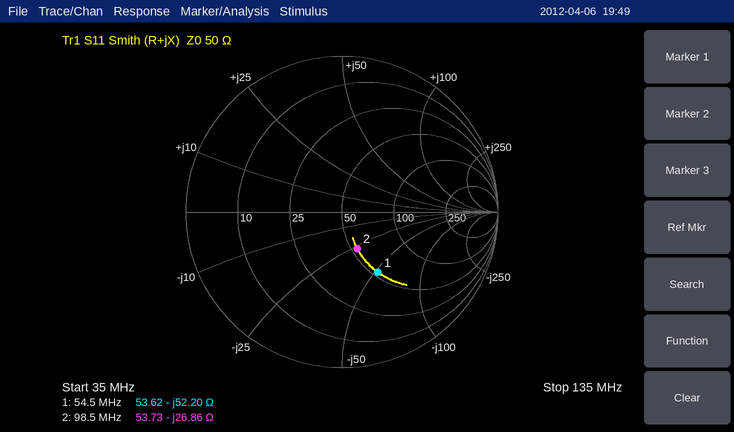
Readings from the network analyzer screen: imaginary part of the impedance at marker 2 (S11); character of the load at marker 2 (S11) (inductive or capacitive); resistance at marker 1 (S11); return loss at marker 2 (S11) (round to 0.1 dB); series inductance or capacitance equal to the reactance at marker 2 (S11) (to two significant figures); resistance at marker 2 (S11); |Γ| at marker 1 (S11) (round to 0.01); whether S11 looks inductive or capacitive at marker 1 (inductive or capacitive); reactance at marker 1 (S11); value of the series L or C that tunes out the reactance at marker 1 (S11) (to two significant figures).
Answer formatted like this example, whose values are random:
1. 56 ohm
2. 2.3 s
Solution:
1. -26.86 Ω
2. capacitive
3. 53.62 Ω
4. 11.9 dB
5. 60 pF
6. 53.73 Ω
7. 0.45
8. capacitive
9. -52.20 Ω
10. 150 nH
